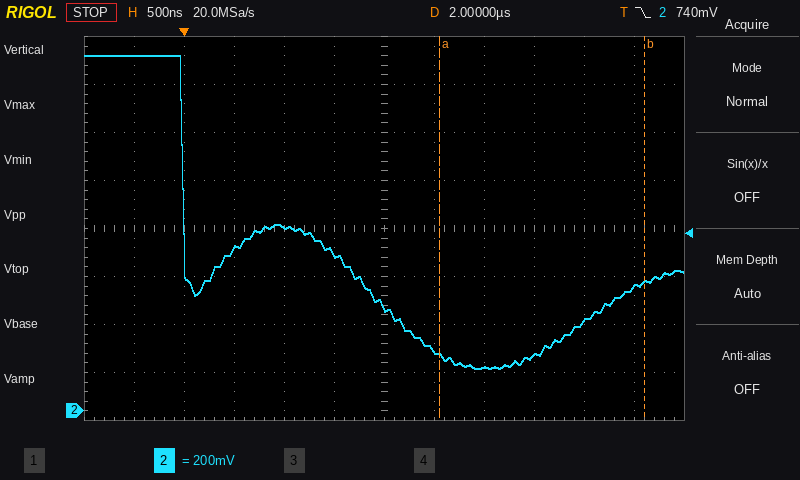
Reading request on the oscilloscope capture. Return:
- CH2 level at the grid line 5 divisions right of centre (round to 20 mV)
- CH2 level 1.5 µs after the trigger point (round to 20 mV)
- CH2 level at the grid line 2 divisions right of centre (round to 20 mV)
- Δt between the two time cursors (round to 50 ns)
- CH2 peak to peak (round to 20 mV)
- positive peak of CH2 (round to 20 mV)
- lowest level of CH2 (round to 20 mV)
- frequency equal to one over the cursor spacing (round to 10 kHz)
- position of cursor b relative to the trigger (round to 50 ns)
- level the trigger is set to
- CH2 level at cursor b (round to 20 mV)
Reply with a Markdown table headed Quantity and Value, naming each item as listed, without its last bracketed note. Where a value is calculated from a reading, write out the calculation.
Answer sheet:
| Quantity | Value |
|---|---|
| CH2 level at the grid line 5 divisions right of centre | 520 mV |
| CH2 level 1.5 µs after the trigger point | 660 mV |
| CH2 level at the grid line 2 divisions right of centre | 180 mV |
| Δt between the two time cursors | 2.05 µs |
| CH2 peak to peak | 1.48 V − (180 mV) = 1.30 V |
| positive peak of CH2 | 1.48 V |
| lowest level of CH2 | 180 mV |
| frequency equal to one over the cursor spacing | 1 / 2.05 µs ≈ 490 kHz |
| position of cursor b relative to the trigger | +4.60 µs |
| level the trigger is set to | 740 mV |
| CH2 level at cursor b | 540 mV |
